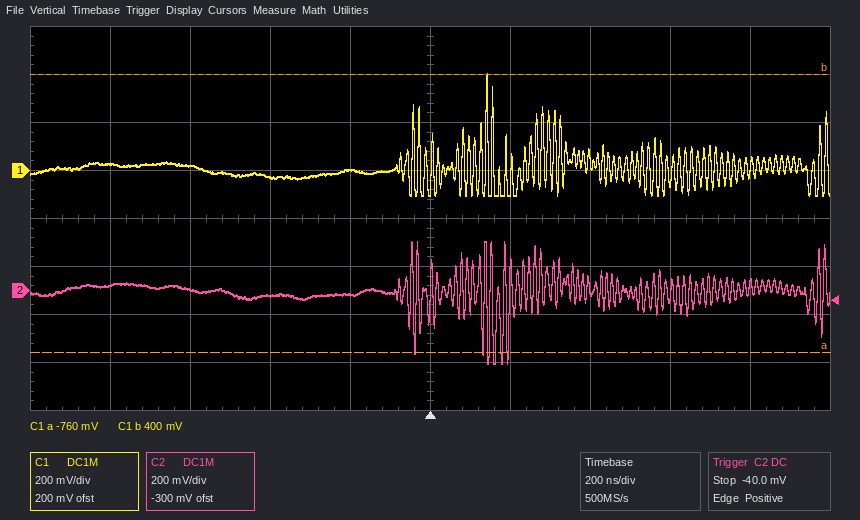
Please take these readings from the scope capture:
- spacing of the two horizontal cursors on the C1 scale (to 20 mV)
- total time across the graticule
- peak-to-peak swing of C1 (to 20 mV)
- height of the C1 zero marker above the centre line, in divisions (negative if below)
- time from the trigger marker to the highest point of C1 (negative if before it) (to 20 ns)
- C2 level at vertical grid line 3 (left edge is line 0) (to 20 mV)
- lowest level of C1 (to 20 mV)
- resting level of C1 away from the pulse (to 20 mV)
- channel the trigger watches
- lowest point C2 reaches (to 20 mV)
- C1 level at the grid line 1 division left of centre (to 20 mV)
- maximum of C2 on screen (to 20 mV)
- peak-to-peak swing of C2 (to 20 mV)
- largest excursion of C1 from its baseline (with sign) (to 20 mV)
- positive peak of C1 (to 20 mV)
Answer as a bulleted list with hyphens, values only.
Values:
- 1.16 V
- 2 µs
- 500 mV
- +1.0 div
- +140 ns
- -20 mV
- -100 mV
- 0 mV
- C2
- -300 mV
- 0 mV
- 200 mV
- 500 mV
- +400 mV
- 400 mV
